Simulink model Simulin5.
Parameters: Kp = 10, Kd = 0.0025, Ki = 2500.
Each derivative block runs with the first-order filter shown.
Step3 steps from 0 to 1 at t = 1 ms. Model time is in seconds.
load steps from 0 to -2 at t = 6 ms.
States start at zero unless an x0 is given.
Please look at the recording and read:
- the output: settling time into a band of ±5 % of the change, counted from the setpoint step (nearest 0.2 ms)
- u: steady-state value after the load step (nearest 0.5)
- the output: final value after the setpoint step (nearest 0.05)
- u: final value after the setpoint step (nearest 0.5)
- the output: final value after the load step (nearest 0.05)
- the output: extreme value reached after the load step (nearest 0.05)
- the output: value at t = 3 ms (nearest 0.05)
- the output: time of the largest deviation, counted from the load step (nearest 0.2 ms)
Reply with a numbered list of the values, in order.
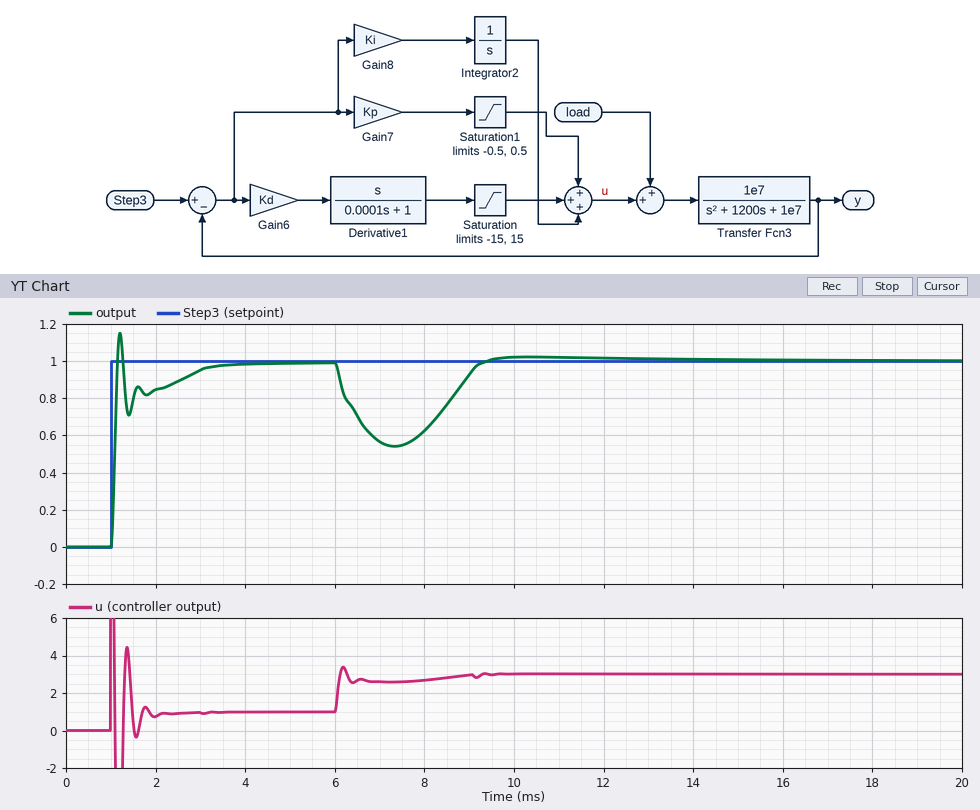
1. 2.0 ms
2. 3.0
3. 1.00
4. 1.0
5. 1.00
6. 0.55
7. 0.95
8. 1.4 ms
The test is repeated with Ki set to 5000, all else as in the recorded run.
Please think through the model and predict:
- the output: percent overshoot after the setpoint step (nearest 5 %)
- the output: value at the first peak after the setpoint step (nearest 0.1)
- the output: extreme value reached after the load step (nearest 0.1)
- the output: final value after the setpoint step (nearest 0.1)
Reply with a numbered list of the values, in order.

1. 15 %
2. 1.2
3. 0.7
4. 1.0
